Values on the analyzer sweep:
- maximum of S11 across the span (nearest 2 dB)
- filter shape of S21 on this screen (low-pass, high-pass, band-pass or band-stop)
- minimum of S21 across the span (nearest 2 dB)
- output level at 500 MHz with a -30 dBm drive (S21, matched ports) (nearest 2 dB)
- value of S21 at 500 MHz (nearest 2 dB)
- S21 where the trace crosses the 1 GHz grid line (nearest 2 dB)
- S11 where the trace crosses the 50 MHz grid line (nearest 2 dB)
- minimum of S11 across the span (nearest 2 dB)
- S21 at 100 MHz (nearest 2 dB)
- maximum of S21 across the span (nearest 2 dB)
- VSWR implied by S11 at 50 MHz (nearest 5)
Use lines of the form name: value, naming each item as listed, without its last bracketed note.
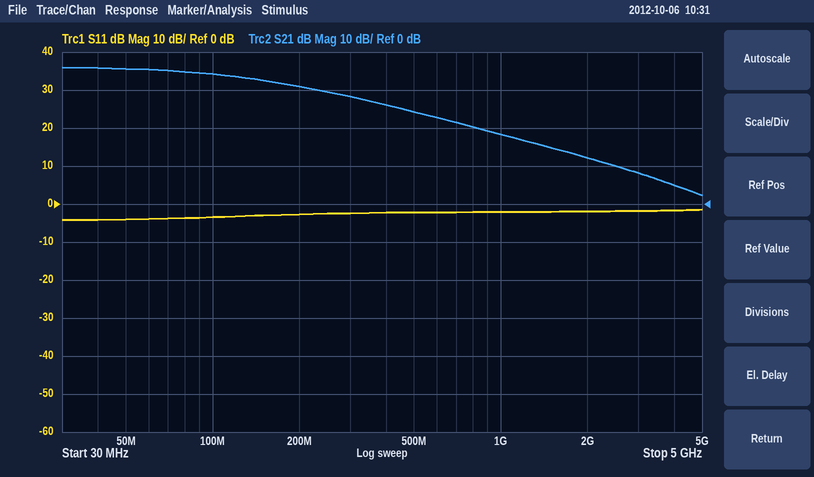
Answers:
maximum of S11 across the span: -2 dB
filter shape of S21 on this screen: low-pass
minimum of S21 across the span: 2 dB
output level at 500 MHz with a -30 dBm drive (S21, matched ports): -6 dBm
value of S21 at 500 MHz: 24 dB
S21 where the trace crosses the 1 GHz grid line: 18 dB
S11 where the trace crosses the 50 MHz grid line: -4 dB
minimum of S11 across the span: -4 dB
S21 at 100 MHz: 34 dB
maximum of S21 across the span: 36 dB
VSWR implied by S11 at 50 MHz: 5
